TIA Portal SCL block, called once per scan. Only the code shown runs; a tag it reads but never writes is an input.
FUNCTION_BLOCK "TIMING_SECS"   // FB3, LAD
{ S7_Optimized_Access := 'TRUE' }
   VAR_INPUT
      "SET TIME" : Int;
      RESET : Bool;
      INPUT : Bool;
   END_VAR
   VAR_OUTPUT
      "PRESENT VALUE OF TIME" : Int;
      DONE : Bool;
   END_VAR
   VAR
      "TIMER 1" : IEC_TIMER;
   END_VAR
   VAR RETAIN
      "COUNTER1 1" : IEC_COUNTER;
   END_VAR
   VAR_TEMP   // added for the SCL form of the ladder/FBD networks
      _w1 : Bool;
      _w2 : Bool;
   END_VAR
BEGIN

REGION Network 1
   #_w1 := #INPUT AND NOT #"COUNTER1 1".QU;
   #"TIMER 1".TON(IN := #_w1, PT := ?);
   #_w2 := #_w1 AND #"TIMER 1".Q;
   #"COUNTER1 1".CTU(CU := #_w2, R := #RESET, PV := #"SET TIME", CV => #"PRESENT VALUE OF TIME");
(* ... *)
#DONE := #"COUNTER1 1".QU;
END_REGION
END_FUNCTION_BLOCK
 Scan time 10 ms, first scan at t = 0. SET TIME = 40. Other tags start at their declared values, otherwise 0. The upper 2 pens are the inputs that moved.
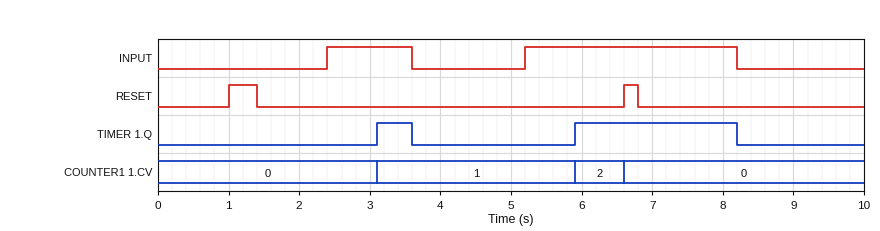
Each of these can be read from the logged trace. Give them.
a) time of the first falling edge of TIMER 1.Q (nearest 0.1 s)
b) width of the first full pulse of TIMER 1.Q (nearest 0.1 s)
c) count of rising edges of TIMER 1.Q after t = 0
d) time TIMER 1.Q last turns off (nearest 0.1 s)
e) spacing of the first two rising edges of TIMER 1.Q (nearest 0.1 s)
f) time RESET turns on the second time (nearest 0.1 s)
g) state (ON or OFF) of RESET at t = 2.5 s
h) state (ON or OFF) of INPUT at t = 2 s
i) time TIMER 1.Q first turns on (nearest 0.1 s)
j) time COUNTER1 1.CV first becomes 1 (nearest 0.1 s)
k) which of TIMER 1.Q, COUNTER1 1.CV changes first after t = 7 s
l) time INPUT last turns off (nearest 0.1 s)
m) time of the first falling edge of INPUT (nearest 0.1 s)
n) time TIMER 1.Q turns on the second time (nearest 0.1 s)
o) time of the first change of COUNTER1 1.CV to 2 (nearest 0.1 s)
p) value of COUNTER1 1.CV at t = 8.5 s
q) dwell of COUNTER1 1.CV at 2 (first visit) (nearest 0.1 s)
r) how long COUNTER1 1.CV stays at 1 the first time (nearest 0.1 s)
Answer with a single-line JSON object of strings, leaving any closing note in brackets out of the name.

{"time of the first falling edge of TIMER 1.Q": "3.6 s", "width of the first full pulse of TIMER 1.Q": "0.5 s", "count of rising edges of TIMER 1.Q after t = 0": "2", "time TIMER 1.Q last turns off": "8.2 s", "spacing of the first two rising edges of TIMER 1.Q": "2.8 s", "time RESET turns on the second time": "6.6 s", "state (ON or OFF) of RESET at t = 2.5 s": "OFF", "state (ON or OFF) of INPUT at t = 2 s": "OFF", "time TIMER 1.Q first turns on": "3.1 s", "time COUNTER1 1.CV first becomes 1": "3.1 s", "which of TIMER 1.Q, COUNTER1 1.CV changes first after t = 7 s": "TIMER 1.Q", "time INPUT last turns off": "8.2 s", "time of the first falling edge of INPUT": "3.6 s", "time TIMER 1.Q turns on the second time": "5.9 s", "time of the first change of COUNTER1 1.CV to 2": "5.9 s", "value of COUNTER1 1.CV at t = 8.5 s": "0", "dwell of COUNTER1 1.CV at 2 (first visit)": "0.7 s", "how long COUNTER1 1.CV stays at 1 the first time": "2.8 s"}
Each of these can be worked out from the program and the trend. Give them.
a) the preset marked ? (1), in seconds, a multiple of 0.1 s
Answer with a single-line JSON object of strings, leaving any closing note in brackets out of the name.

{"the preset marked ? (1), in seconds, a multiple of 0.1 s": "0.7 s"}
